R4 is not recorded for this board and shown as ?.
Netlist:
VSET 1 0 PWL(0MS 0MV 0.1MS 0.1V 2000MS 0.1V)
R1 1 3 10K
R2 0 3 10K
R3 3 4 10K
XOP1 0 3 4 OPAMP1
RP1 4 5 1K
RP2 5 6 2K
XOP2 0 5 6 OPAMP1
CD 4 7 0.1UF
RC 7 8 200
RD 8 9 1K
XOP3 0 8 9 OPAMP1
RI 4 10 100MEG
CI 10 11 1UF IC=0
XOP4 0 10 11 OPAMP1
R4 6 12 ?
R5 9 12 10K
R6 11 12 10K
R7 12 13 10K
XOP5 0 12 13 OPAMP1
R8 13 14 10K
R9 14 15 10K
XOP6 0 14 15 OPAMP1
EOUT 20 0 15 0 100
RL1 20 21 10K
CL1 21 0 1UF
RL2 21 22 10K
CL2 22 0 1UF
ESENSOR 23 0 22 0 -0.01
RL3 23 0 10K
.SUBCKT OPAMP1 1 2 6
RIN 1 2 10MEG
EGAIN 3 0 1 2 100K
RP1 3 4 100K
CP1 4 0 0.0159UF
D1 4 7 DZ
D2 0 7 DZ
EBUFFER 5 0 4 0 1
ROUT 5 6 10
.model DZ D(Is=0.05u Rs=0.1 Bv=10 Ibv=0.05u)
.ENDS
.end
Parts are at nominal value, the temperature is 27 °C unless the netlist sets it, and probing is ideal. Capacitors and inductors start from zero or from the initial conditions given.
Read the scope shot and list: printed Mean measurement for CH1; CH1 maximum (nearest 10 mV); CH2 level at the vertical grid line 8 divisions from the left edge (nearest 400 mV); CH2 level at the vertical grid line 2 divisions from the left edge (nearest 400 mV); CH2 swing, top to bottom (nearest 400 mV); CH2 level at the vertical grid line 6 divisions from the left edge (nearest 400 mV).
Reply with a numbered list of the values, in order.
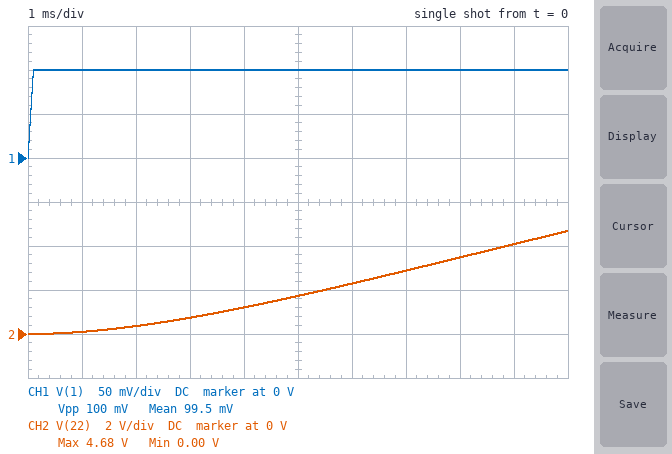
1. 99.5 mV
2. 100 mV
3. 3.6 V
4. 400 mV
5. 4.8 V
6. 2.4 V
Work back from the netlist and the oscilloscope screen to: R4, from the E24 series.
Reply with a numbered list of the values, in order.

1. 9.1 kΩ
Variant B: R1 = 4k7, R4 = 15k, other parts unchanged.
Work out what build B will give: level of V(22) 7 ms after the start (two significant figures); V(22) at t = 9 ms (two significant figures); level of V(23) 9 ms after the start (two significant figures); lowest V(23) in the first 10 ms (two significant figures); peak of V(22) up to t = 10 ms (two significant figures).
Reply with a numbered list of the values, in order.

1. 3.7 V
2. 5.3 V
3. -53 mV
4. -61 mV
5. 6.1 V
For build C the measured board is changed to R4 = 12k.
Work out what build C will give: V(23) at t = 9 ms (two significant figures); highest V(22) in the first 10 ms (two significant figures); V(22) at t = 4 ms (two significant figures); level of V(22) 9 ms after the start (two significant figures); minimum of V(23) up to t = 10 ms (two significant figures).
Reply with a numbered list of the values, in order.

1. -31 mV
2. 3.6 V
3. 920 mV
4. 3.1 V
5. -36 mV
